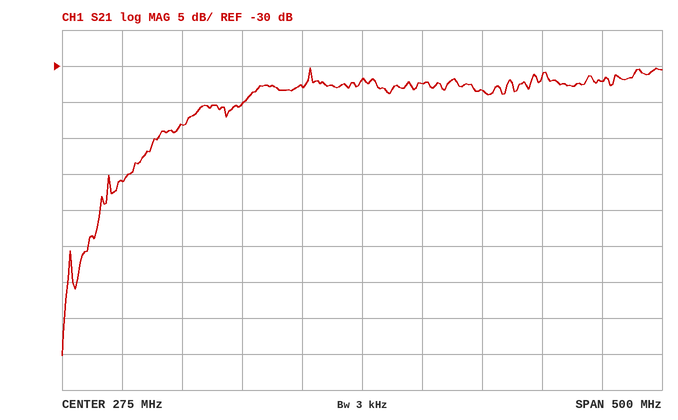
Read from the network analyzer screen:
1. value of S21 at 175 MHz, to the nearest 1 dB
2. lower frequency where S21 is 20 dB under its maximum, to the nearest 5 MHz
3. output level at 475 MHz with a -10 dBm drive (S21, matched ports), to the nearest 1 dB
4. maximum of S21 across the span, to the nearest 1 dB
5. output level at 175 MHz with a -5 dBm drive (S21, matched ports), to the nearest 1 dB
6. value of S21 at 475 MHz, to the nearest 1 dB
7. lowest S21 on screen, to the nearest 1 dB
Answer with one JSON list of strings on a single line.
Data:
["-35 dB", "55 MHz", "-42 dBm", "-30 dB", "-40 dBm", "-32 dB", "-70 dB"]
